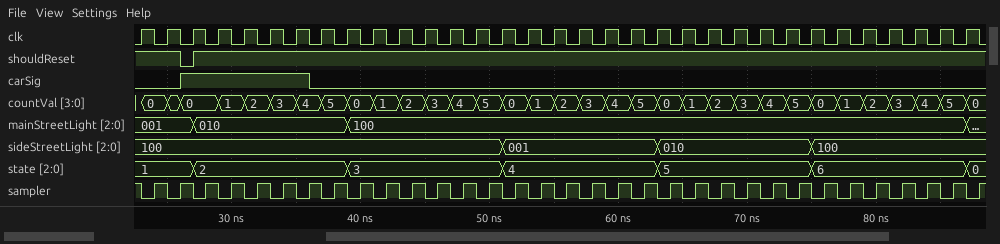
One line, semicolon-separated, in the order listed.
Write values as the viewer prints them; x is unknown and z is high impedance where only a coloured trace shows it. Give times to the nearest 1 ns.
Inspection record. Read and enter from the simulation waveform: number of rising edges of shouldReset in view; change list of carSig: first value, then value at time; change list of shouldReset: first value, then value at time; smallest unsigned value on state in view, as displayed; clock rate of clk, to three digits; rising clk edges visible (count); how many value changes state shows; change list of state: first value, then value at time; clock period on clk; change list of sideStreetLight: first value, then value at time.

1; 0, 1 at 26 ns, 0 at 36 ns; 1, 0 at 26 ns, 1 at 27 ns; 0; 500 MHz; 33; 6; 1, 2 at 27 ns, 3 at 39 ns, 4 at 51 ns, 5 at 63 ns, 6 at 75 ns, 0 at 87 ns; 2 ns; 100, 001 at 51 ns, 010 at 63 ns, 100 at 75 ns
